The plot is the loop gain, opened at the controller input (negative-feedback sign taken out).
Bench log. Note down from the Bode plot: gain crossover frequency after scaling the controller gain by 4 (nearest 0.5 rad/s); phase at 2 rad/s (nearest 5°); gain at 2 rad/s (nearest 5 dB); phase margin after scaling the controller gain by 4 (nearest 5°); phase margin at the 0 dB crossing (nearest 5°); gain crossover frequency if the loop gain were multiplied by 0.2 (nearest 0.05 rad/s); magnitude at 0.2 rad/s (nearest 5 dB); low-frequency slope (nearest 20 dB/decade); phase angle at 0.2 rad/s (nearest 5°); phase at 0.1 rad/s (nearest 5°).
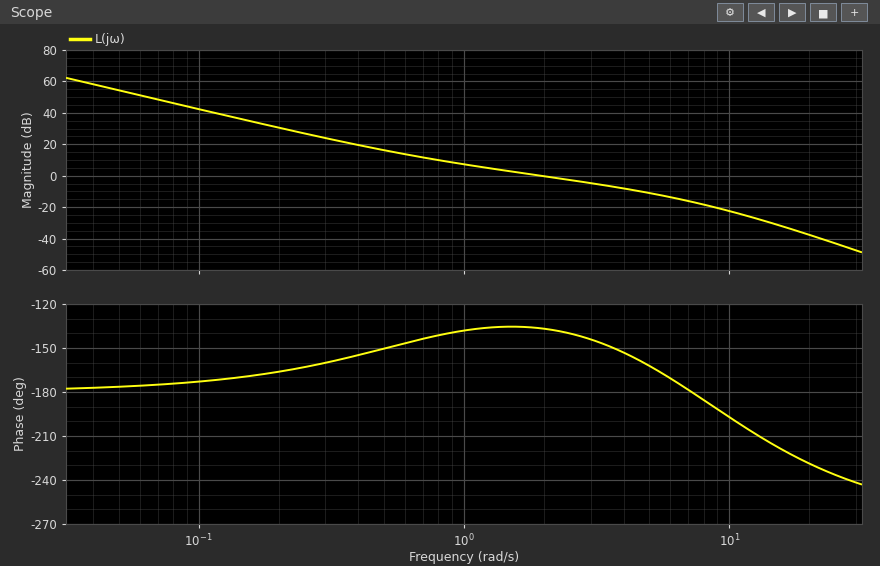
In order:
5.5 rad/s
-135°
0 dB
15°
45°
0.60 rad/s
30 dB
-40 dB/decade
-165°
-175°
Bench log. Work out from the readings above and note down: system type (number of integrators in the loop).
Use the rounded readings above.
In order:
2
